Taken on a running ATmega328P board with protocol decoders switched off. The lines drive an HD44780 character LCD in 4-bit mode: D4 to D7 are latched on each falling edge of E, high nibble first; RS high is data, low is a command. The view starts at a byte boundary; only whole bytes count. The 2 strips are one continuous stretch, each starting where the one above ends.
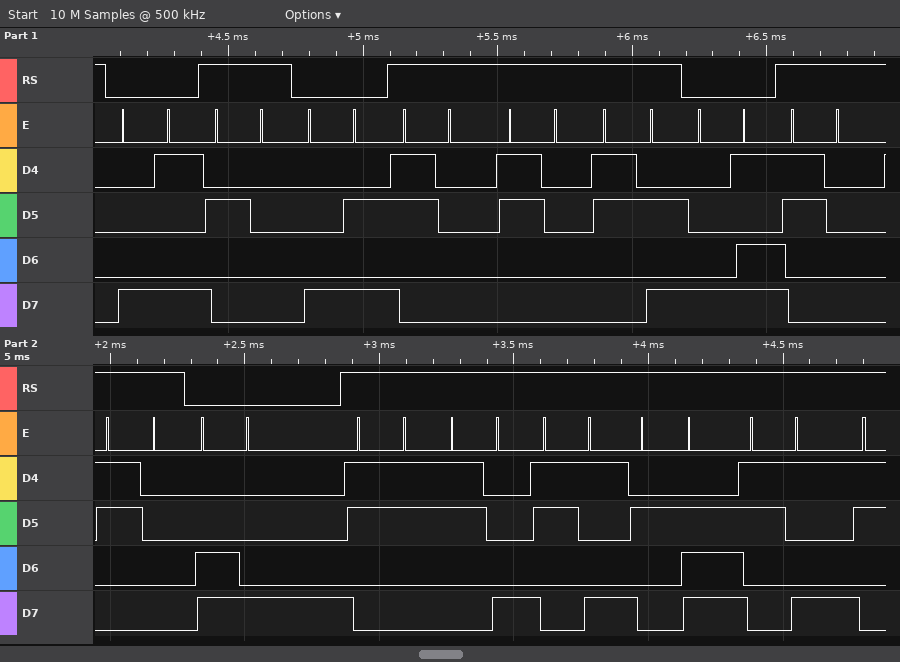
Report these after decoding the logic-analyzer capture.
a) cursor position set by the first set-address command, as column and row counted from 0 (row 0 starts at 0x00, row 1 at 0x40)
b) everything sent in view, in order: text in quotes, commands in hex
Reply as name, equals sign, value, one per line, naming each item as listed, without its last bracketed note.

cursor position set by the first set-address command, as column and row counted from 0 = column 9, row 0
everything sent in view, in order: text in quotes, commands in hex = 0x89 " " 0x8A "00:" 0x8D "00" 0xC8 "389.9"
